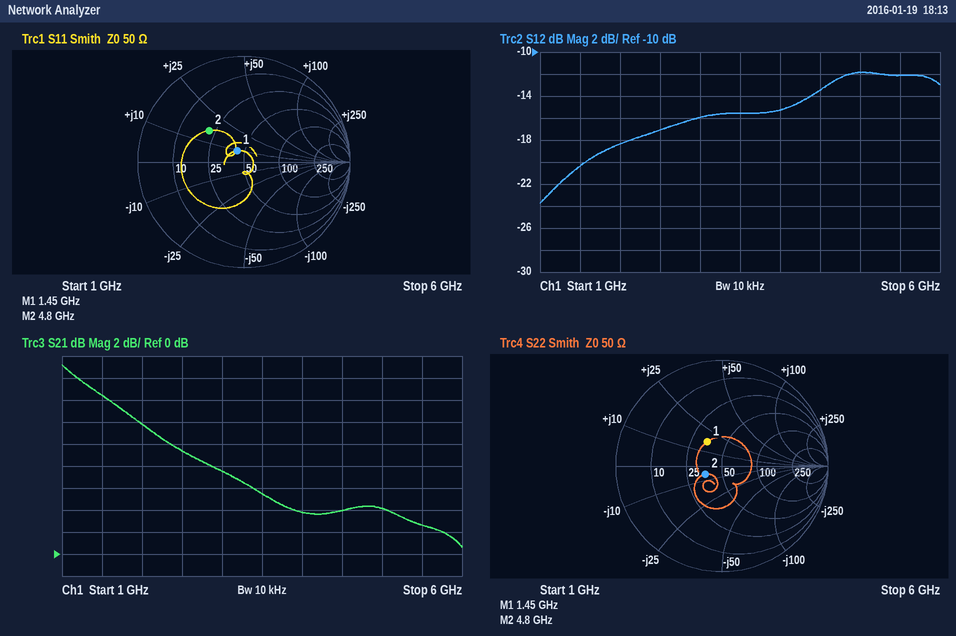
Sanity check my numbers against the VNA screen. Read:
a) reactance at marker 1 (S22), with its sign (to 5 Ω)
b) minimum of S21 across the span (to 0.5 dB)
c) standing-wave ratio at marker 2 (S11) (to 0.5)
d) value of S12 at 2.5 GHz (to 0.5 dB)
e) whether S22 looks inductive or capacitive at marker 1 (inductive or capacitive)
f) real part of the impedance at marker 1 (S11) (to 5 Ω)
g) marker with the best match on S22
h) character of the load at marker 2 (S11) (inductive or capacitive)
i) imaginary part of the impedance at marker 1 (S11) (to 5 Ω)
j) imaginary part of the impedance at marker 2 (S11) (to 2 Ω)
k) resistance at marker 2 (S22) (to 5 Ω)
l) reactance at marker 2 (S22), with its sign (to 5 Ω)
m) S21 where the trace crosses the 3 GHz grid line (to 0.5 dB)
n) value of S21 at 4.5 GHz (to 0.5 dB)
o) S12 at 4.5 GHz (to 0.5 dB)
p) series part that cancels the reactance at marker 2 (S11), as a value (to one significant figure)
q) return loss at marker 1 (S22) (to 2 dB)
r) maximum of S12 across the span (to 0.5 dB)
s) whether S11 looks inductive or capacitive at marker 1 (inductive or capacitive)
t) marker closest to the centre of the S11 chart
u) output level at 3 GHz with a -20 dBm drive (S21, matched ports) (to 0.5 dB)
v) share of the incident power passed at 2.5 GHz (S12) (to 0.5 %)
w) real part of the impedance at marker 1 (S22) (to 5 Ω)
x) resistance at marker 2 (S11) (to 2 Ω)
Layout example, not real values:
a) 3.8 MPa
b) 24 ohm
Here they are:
a) +15 Ω
b) 0.5 dB
c) 2.5
d) -17.0 dB
e) inductive
f) 45 Ω
g) marker 2
h) inductive
i) +10 Ω
j) +16 Ω
k) 35 Ω
l) -5 Ω
m) 7.5 dB
n) 4.0 dB
o) -13.5 dB
p) 2 pF
q) 12 dB
r) -12.0 dB
s) inductive
t) marker 1
u) -12.5 dBm
v) 2.0 %
w) 35 Ω
x) 22 Ω
